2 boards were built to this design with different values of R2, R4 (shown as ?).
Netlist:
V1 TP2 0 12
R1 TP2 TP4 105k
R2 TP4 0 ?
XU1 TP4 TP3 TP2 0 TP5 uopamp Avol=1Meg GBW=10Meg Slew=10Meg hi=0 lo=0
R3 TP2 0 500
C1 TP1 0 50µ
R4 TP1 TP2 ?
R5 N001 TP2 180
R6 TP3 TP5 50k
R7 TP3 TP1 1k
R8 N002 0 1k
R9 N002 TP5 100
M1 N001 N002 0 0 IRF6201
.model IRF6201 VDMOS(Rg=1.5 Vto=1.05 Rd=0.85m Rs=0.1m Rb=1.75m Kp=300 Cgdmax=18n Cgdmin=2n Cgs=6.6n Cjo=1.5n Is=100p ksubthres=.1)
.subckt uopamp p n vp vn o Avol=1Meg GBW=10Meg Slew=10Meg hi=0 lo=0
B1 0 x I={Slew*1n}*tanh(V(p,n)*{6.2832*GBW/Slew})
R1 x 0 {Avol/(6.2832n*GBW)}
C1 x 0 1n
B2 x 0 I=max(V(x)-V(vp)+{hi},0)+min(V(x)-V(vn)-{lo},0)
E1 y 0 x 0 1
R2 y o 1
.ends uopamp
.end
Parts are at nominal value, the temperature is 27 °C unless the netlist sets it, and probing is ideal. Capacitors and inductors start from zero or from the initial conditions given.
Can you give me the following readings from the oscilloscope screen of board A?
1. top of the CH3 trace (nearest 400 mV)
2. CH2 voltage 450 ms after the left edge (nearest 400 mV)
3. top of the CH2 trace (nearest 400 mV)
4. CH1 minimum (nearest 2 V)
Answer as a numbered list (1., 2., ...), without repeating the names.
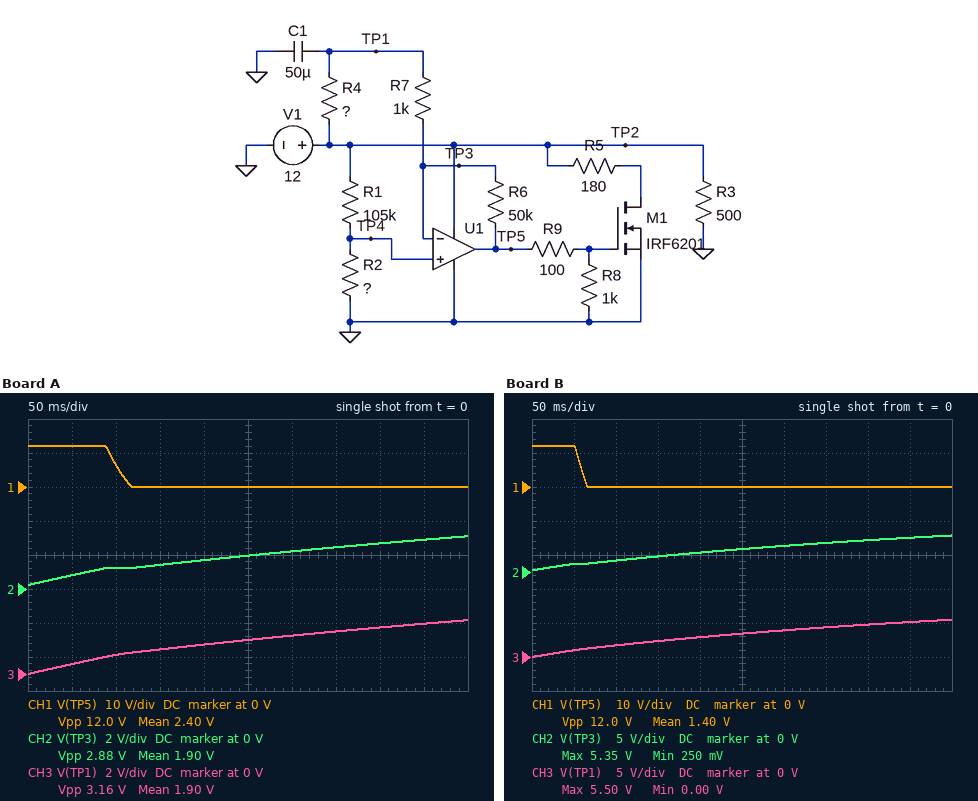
1. 3.2 V
2. 2.8 V
3. 3.2 V
4. 0 V
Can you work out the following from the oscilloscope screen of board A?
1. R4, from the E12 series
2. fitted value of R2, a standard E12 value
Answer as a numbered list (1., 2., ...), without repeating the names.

1. 33 kΩ
2. 12 kΩ
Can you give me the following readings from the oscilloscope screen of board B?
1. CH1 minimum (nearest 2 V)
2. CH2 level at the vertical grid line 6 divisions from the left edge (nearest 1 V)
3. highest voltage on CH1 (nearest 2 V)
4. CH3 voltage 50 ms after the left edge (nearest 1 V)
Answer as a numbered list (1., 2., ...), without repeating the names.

1. 0 V
2. 4 V
3. 12 V
4. 1 V
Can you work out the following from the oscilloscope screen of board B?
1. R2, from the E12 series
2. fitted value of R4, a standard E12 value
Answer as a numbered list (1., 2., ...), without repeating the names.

1. 12 kΩ
2. 15 kΩ
